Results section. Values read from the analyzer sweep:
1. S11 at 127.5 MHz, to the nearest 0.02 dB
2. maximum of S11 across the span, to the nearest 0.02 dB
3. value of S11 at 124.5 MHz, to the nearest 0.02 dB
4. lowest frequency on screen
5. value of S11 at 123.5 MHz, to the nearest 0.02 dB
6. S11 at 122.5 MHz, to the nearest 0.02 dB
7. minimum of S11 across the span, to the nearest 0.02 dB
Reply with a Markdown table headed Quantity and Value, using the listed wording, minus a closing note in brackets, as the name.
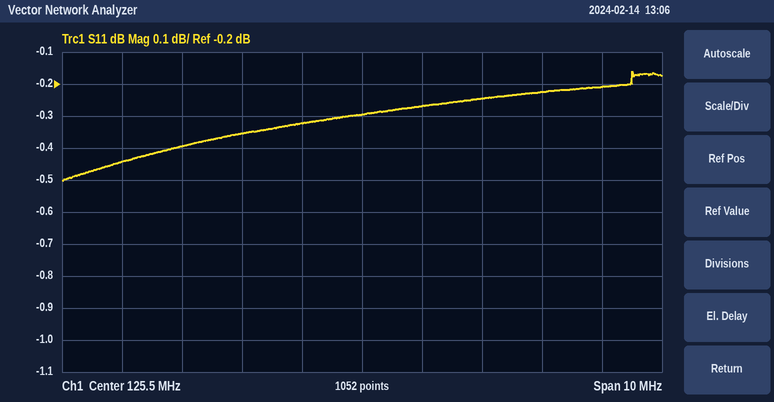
| Quantity | Value |
|---|---|
| S11 at 127.5 MHz, to the nearest 0.02 dB | -0.24 dB |
| maximum of S11 across the span, to the nearest 0.02 dB | -0.16 dB |
| value of S11 at 124.5 MHz, to the nearest 0.02 dB | -0.32 dB |
| lowest frequency on screen | 120.5 MHz |
| value of S11 at 123.5 MHz, to the nearest 0.02 dB | -0.36 dB |
| S11 at 122.5 MHz, to the nearest 0.02 dB | -0.40 dB |
| minimum of S11 across the span, to the nearest 0.02 dB | -0.50 dB |
